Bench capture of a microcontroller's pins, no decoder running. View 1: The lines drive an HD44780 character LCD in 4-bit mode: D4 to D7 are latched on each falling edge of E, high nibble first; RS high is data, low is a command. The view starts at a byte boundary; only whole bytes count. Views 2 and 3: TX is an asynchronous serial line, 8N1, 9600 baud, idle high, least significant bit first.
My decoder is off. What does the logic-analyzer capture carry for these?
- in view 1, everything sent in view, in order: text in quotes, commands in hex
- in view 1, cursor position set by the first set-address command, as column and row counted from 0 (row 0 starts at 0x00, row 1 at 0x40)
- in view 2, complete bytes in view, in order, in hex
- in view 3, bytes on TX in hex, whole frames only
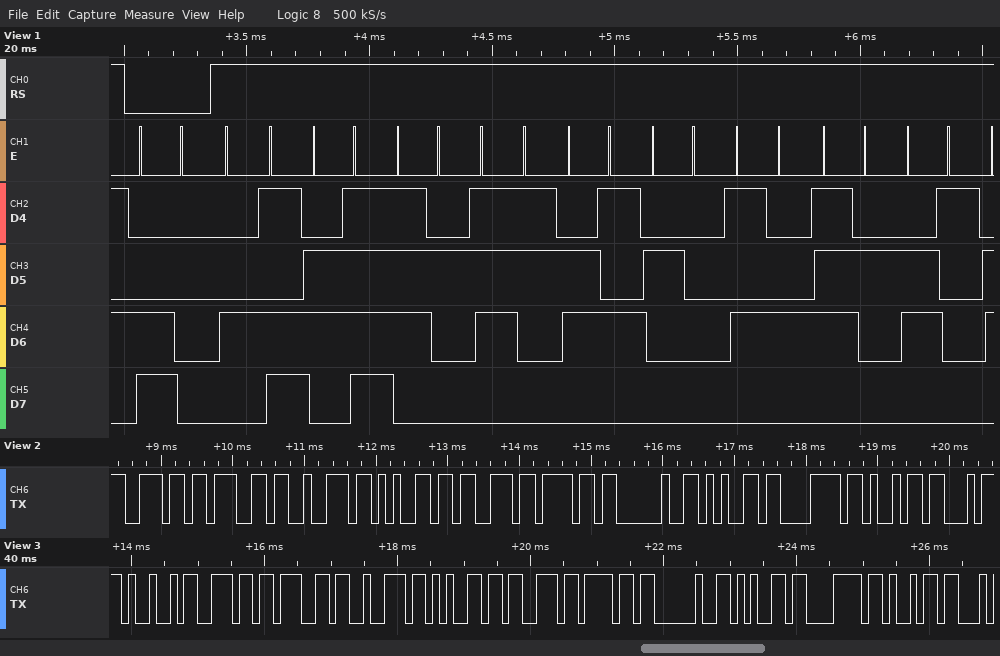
0xC0 "Morse Tra"
column 0, row 1
6E 67 72 65 73 6F 20 65 78 69
49 6E 67 72 65 73 6F 20 65 78 69
